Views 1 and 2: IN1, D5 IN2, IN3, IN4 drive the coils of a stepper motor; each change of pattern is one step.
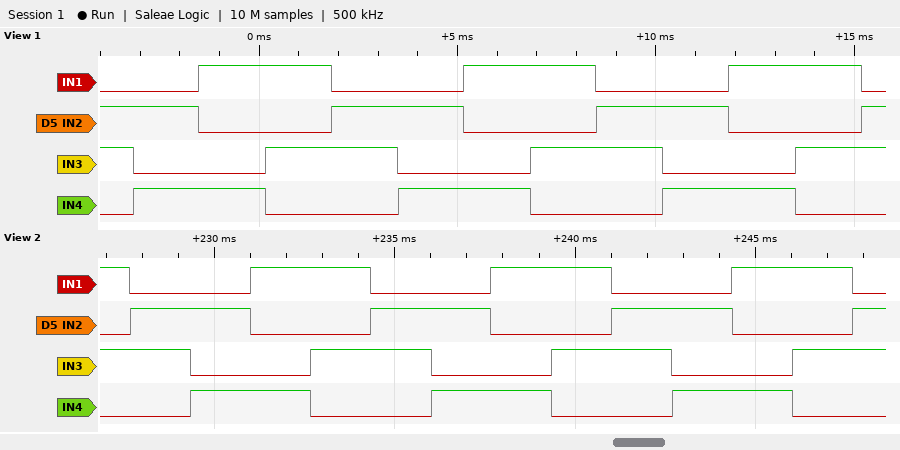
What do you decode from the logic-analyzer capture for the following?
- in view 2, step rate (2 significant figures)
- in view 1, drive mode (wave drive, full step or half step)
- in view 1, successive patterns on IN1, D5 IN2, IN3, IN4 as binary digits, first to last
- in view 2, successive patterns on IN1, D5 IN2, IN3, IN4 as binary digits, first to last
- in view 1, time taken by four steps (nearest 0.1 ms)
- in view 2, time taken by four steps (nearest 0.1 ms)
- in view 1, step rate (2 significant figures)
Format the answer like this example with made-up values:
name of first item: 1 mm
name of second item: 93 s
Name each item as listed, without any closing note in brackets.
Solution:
in view 2, step rate: 600 steps/s
in view 1, drive mode: full step
in view 1, successive patterns on IN1, D5 IN2, IN3, IN4 as binary digits, first to last: 0110 0101 1001 1010 0110 0101 1001 1010 0110 0101 1001 1010 0110
in view 2, successive patterns on IN1, D5 IN2, IN3, IN4 as binary digits, first to last: 1010 0110 0101 1001 1010 0110 0101 1001 1010 0110 0101 1001 1010 0110
in view 1, time taken by four steps: 6.7 ms
in view 2, time taken by four steps: 6.7 ms
in view 1, step rate: 600 steps/s
